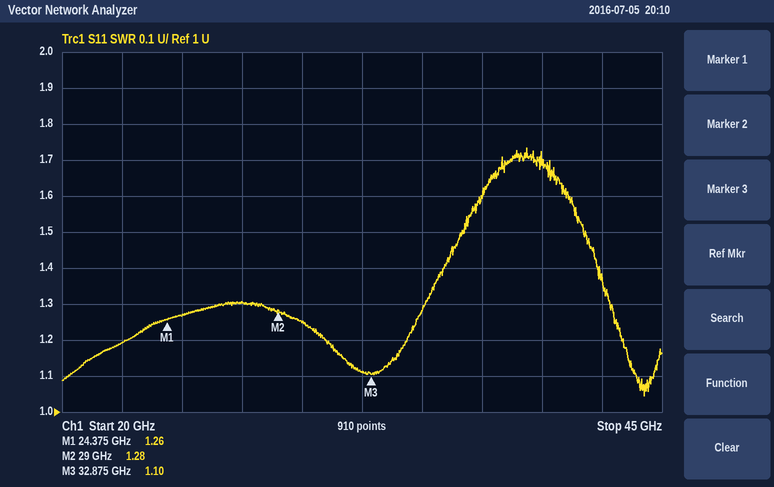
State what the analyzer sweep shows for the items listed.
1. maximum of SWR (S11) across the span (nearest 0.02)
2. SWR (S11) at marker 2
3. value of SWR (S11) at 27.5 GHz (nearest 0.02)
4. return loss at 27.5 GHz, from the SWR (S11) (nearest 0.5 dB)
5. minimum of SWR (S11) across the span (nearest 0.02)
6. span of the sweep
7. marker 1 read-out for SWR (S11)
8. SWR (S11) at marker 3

1.74
1.28
1.30
17.5 dB
1.04
25 GHz
1.26
1.10
